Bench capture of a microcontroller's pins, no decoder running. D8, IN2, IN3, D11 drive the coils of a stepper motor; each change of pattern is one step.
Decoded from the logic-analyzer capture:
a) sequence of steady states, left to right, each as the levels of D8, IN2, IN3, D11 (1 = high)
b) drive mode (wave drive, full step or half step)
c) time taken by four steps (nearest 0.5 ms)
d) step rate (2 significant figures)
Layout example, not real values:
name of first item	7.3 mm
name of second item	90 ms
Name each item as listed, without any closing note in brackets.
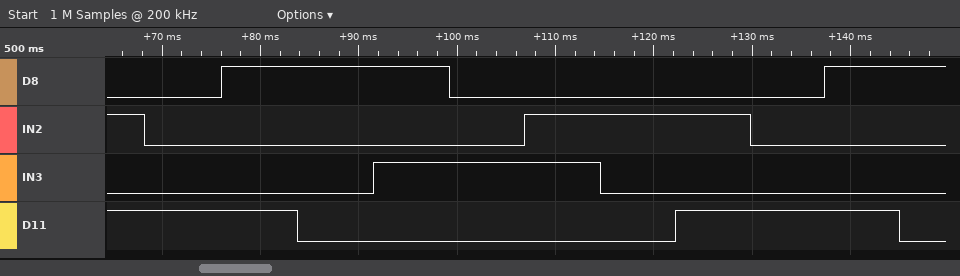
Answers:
sequence of steady states, left to right, each as the levels of D8, IN2, IN3, D11	0101 0001 1001 1000 1010 0010 0110 0100 0101 0001 1001 1000
drive mode	half step
time taken by four steps	31.0 ms
step rate	130 steps/s
